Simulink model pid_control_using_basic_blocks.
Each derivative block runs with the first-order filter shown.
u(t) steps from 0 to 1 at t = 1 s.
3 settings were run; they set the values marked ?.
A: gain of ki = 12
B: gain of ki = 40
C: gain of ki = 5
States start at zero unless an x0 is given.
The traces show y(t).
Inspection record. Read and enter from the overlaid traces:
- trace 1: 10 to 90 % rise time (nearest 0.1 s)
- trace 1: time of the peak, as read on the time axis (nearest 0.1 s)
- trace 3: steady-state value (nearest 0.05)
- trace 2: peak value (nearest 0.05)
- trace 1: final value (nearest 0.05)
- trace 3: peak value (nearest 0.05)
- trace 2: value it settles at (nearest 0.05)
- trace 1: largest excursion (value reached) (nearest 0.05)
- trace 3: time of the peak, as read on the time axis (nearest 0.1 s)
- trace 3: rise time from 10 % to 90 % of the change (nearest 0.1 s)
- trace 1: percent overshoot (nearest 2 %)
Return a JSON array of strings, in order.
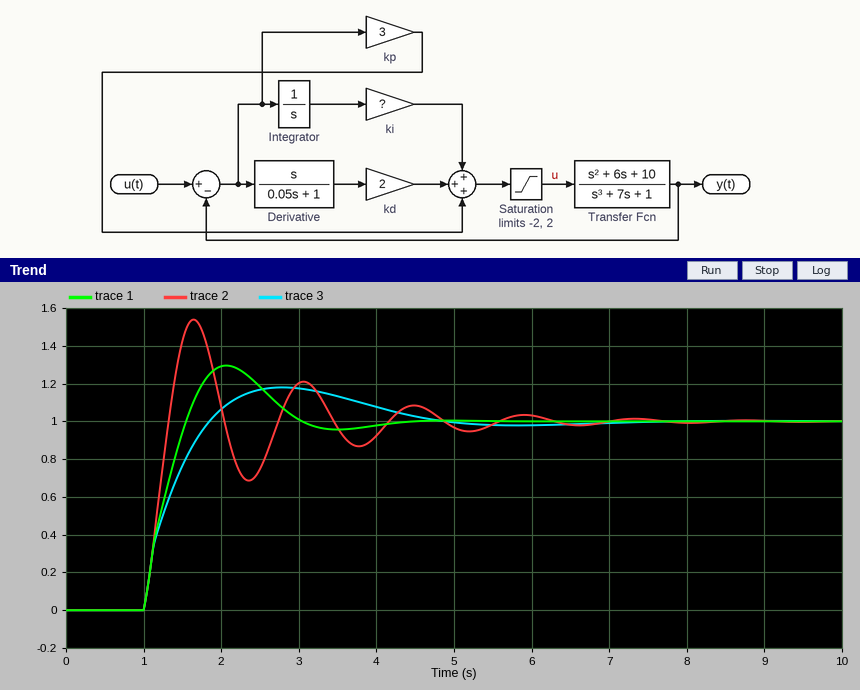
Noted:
["0.4 s", "2.1 s", "1.00", "1.55", "1.00", "1.20", "1.00", "1.30", "2.8 s", "0.6 s", "30 %"]
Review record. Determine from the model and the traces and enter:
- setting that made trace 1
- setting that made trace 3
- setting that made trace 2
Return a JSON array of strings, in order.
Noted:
["A", "C", "B"]
